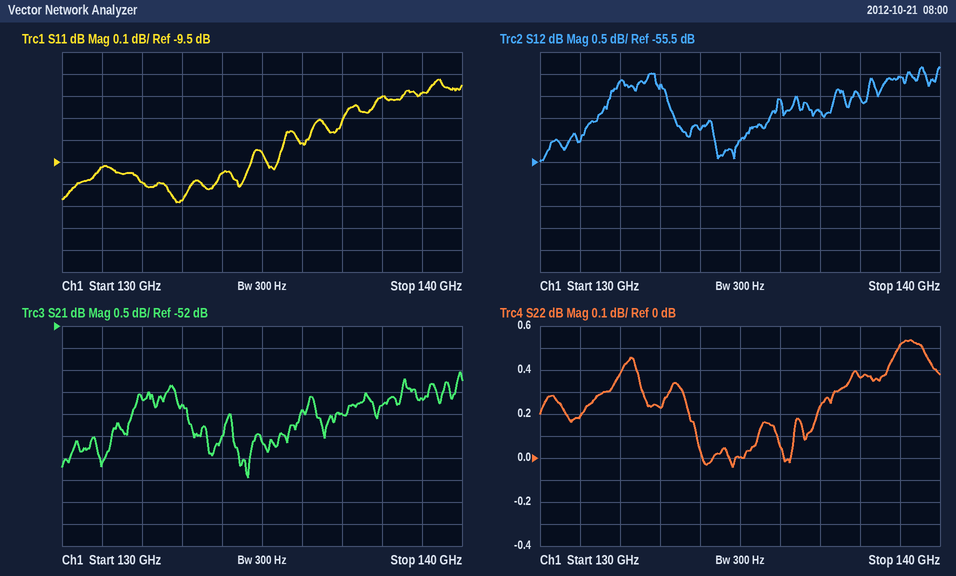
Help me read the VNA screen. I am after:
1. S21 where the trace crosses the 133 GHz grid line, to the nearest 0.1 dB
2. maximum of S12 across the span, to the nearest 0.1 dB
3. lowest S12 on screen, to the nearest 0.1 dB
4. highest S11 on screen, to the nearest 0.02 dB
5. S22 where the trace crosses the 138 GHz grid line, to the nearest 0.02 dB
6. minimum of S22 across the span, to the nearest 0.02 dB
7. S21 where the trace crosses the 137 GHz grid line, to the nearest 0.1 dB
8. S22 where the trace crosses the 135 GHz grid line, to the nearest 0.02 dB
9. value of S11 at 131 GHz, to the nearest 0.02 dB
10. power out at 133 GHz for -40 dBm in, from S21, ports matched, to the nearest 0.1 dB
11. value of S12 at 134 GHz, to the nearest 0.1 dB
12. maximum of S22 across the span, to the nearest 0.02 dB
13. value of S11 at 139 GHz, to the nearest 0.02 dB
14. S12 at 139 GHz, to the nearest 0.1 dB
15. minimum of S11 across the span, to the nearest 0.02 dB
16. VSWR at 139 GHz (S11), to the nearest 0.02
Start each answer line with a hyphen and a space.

- -53.8 dB
- -53.3 dB
- -55.5 dB
- -9.12 dB
- 0.36 dB
- -0.04 dB
- -54.0 dB
- 0.00 dB
- -9.52 dB
- -93.8 dBm
- -54.8 dB
- 0.54 dB
- -9.18 dB
- -53.6 dB
- -9.68 dB
- 2.06
